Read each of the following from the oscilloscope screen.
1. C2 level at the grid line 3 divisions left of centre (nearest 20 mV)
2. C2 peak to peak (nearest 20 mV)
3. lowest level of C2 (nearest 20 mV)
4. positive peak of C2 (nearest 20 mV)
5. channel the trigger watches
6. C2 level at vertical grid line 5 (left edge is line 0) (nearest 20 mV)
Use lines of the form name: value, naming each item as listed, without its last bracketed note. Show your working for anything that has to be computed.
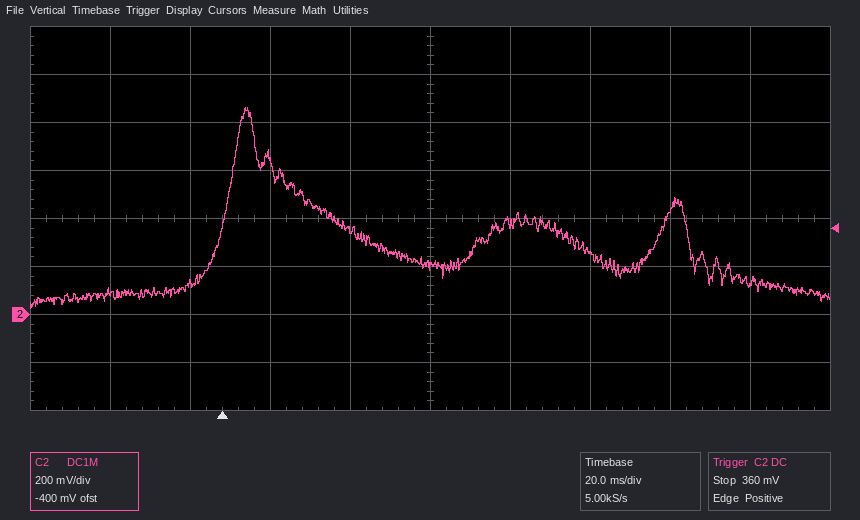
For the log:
C2 level at the grid line 3 divisions left of centre: 120 mV
C2 peak to peak: 860 mV − (20 mV) = 840 mV
lowest level of C2: 20 mV
positive peak of C2: 860 mV
channel the trigger watches: C2
C2 level at vertical grid line 5 (left edge is line 0): 200 mV
